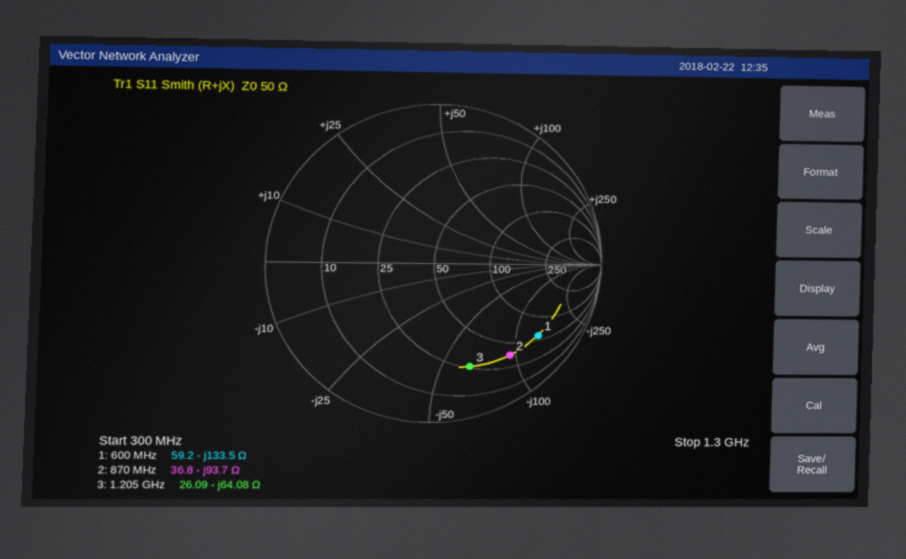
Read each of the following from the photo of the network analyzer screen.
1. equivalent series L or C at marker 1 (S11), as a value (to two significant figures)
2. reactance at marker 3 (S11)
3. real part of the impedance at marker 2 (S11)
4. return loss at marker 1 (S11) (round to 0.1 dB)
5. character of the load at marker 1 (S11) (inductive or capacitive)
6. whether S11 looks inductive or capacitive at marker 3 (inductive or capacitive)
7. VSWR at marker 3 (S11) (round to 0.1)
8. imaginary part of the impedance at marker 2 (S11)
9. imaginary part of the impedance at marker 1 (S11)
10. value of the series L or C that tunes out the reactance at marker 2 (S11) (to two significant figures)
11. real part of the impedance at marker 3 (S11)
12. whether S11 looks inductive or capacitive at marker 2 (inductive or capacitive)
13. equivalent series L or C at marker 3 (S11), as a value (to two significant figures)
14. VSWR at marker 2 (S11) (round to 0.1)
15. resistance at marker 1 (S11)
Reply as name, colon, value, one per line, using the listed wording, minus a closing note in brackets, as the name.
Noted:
equivalent series L or C at marker 1 (S11), as a value: 2.0 pF
reactance at marker 3: -64.08 Ω
real part of the impedance at marker 2: 36.8 Ω
return loss at marker 1 (S11): 2.2 dB
character of the load at marker 1 (S11): capacitive
whether S11 looks inductive or capacitive at marker 3: capacitive
VSWR at marker 3 (S11): 5.4
imaginary part of the impedance at marker 2: -93.7 Ω
imaginary part of the impedance at marker 1: -133.5 Ω
value of the series L or C that tunes out the reactance at marker 2 (S11): 17 nH
real part of the impedance at marker 3: 26.09 Ω
whether S11 looks inductive or capacitive at marker 2: capacitive
equivalent series L or C at marker 3 (S11), as a value: 2.1 pF
VSWR at marker 2 (S11): 6.7
resistance at marker 1: 59.2 Ω
